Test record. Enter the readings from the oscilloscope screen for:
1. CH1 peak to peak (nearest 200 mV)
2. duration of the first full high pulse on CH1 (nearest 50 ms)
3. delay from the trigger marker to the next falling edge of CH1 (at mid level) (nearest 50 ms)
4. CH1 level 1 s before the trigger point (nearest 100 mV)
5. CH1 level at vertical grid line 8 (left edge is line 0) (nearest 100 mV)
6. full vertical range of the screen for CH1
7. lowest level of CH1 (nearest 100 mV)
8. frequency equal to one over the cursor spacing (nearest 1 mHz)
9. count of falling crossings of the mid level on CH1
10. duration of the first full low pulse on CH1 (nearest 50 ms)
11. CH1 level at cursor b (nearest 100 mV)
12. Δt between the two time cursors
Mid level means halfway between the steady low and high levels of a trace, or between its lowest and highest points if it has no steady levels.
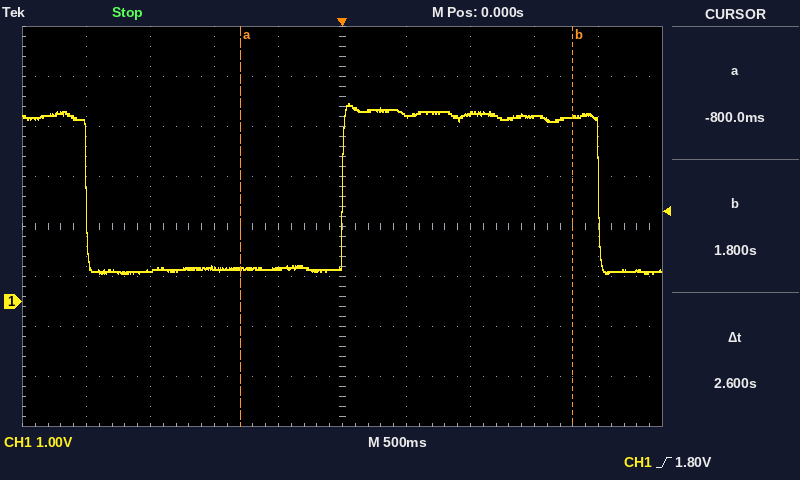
3.4 V
2.00 s
2.00 s
700 mV
3.7 V
8 V
600 mV
385 mHz
2
2.00 s
3.7 V
2.6 s
